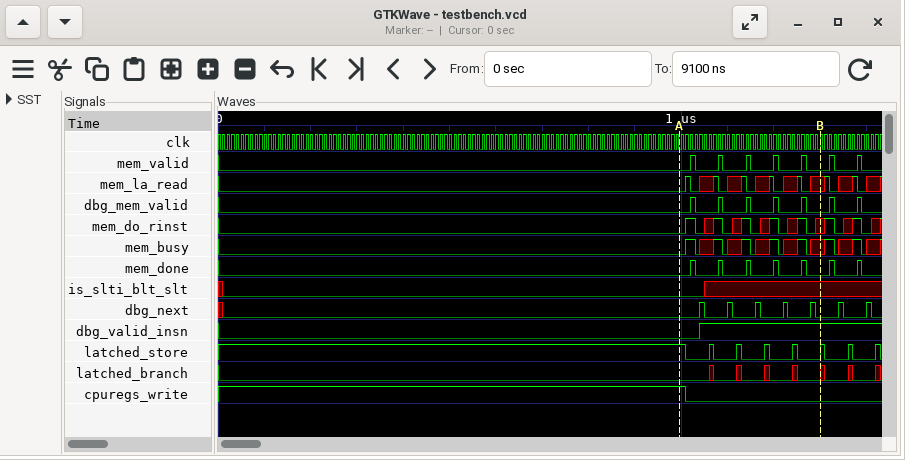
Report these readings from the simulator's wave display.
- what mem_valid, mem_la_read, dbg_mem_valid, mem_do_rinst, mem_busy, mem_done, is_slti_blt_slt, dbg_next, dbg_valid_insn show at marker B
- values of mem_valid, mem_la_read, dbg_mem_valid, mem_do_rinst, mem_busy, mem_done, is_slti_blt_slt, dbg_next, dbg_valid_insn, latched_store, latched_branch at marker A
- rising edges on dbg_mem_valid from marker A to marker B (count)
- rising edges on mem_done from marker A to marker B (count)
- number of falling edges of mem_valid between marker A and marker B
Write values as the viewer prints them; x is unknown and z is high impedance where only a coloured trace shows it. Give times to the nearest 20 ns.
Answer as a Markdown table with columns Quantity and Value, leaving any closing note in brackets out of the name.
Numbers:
| Quantity | Value |
|---|---|
| what mem_valid, mem_la_read, dbg_mem_valid, mem_do_rinst, mem_busy, mem_done, is_slti_blt_slt, dbg_next, dbg_valid_insn show at marker B | mem_valid=0, mem_la_read=x, dbg_mem_valid=0, mem_do_rinst=x, mem_busy=x, mem_done=0, is_slti_blt_slt=x, dbg_next=0, dbg_valid_insn=1 |
| values of mem_valid, mem_la_read, dbg_mem_valid, mem_do_rinst, mem_busy, mem_done, is_slti_blt_slt, dbg_next, dbg_valid_insn, latched_store, latched_branch at marker A | mem_valid=0, mem_la_read=0, dbg_mem_valid=0, mem_do_rinst=0, mem_busy=0, mem_done=0, is_slti_blt_slt=0, dbg_next=0, dbg_valid_insn=0, latched_store=1, latched_branch=0 |
| rising edges on dbg_mem_valid from marker A to marker B | 5 |
| rising edges on mem_done from marker A to marker B | 5 |
| number of falling edges of mem_valid between marker A and marker B | 5 |
